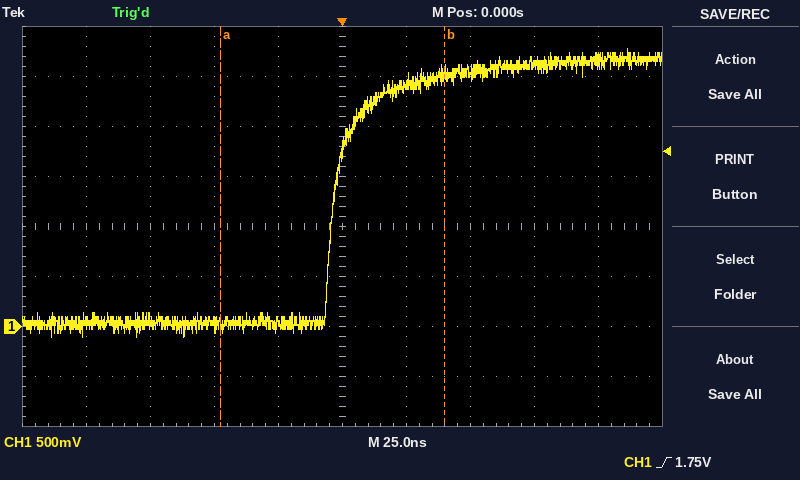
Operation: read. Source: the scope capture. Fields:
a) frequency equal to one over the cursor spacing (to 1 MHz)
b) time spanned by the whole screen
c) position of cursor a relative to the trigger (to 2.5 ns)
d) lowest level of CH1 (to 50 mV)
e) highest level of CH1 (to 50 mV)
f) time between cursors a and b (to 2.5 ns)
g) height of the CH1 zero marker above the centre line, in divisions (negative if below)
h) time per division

11 MHz
250 ns
-47.5 ns
-100 mV
2.80 V
87.5 ns
-2.0 div
25 ns
